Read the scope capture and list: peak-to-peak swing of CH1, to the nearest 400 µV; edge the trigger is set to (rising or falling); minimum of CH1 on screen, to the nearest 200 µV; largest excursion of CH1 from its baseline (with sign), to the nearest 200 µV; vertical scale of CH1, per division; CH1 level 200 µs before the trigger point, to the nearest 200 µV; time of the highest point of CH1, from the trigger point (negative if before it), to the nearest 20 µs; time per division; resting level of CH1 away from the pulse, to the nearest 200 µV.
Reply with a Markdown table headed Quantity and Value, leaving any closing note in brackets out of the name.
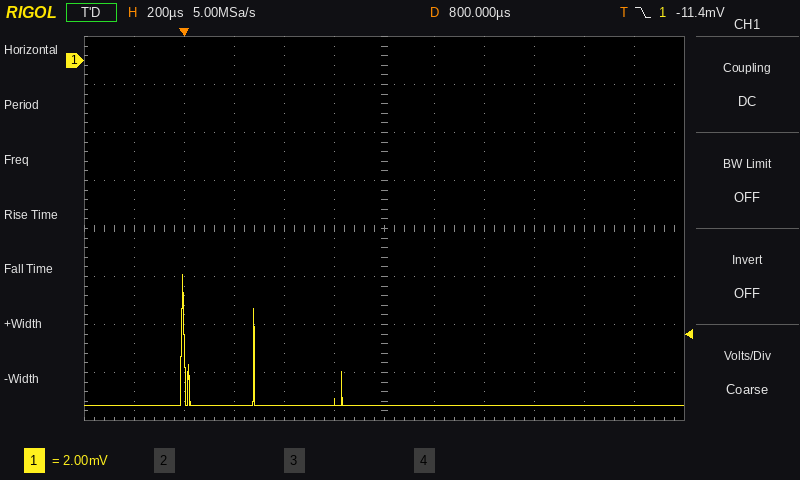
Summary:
| Quantity | Value |
|---|---|
| peak-to-peak swing of CH1, to the nearest 400 µV | 5.6 mV |
| edge the trigger is set to | falling |
| minimum of CH1 on screen, to the nearest 200 µV | -14.4 mV |
| largest excursion of CH1 from its baseline (with sign), to the nearest 200 µV | +5.4 mV |
| vertical scale of CH1, per division | 2 mV |
| CH1 level 200 µs before the trigger point, to the nearest 200 µV | -14.4 mV |
| time of the highest point of CH1, from the trigger point (negative if before it), to the nearest 20 µs | 0 µs |
| time per division | 200 µs |
| resting level of CH1 away from the pulse, to the nearest 200 µV | -14.4 mV |
